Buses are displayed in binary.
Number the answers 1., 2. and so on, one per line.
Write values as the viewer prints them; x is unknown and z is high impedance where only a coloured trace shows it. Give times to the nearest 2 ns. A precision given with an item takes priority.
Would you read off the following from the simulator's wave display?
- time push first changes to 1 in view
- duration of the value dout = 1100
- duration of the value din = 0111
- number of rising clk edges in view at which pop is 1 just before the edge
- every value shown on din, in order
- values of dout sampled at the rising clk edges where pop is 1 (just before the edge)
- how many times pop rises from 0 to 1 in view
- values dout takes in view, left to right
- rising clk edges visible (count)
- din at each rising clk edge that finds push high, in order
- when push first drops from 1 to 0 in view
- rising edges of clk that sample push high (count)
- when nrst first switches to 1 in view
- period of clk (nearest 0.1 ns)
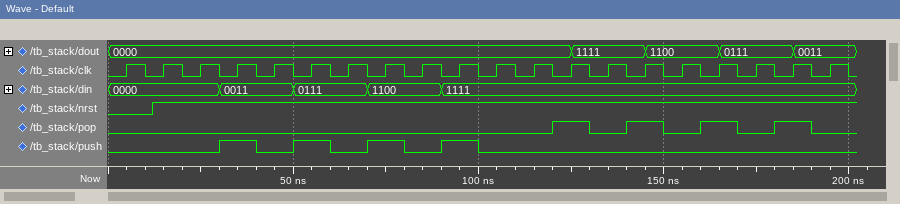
1. 30 ns
2. 20 ns
3. 20 ns
4. 4
5. 0000, 0011, 0111, 1100, 1111
6. 0000, 1111, 1100, 0111
7. 4
8. 0000, 1111, 1100, 0111, 0011
9. 20
10. 0011, 0111, 1100, 1111
11. 40 ns
12. 4
13. 12 ns
14. 10 ns
